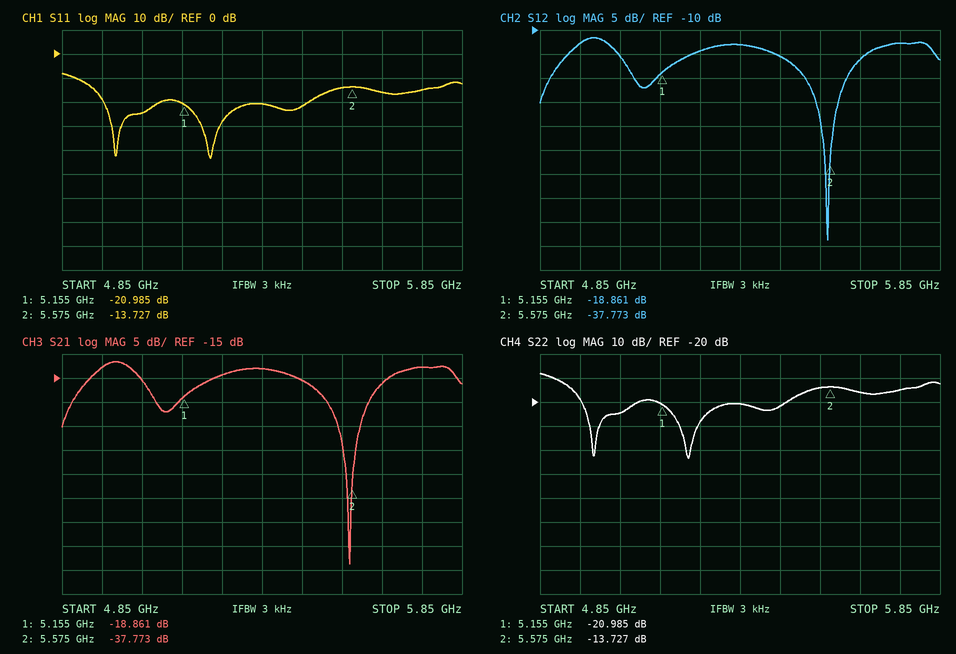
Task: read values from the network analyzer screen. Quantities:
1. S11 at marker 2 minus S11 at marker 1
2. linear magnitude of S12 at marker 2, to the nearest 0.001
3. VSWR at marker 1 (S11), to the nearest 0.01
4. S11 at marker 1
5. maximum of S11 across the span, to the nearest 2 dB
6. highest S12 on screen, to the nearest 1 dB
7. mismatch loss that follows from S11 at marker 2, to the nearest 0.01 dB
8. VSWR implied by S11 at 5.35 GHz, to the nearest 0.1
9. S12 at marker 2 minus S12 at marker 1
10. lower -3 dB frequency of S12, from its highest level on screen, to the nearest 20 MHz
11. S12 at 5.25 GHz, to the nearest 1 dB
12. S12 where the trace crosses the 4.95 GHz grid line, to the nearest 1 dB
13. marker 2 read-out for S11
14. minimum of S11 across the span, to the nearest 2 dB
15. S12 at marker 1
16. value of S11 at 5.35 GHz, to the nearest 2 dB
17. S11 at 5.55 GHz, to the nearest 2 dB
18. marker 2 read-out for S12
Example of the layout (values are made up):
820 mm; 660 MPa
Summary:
7.258 dB; 0.013; 1.20; -20.985 dB; -8 dB; -12 dB; 0.19 dB; 1.2; -18.912 dB; 4.92 GHz; -14 dB; -13 dB; -13.727 dB; -44 dB; -18.861 dB; -20 dB; -14 dB; -37.773 dB
